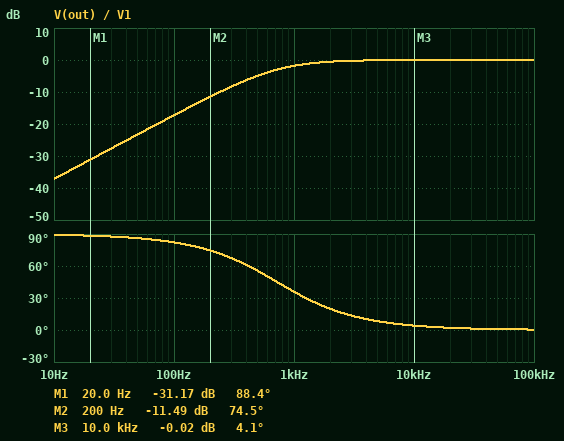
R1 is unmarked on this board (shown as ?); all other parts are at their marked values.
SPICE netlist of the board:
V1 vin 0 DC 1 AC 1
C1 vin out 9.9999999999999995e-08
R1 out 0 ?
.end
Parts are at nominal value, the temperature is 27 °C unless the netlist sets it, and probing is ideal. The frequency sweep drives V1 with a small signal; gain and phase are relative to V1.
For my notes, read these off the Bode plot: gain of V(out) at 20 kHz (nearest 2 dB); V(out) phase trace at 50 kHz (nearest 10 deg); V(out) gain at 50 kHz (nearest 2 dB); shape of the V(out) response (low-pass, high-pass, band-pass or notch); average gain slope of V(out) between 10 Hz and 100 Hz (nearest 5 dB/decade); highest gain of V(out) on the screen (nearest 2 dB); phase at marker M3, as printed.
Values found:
0 dB
0 deg
0 dB
high-pass
20 dB/decade
0 dB
4.1 deg
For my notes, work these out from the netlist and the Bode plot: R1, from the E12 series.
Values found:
2.2 kΩ
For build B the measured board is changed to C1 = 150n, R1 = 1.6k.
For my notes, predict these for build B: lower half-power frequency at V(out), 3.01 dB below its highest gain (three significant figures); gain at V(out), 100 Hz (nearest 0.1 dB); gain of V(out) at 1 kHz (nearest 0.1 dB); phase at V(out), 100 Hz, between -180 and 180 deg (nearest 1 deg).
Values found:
663 Hz
-16.5 dB
-1.6 dB
81 deg
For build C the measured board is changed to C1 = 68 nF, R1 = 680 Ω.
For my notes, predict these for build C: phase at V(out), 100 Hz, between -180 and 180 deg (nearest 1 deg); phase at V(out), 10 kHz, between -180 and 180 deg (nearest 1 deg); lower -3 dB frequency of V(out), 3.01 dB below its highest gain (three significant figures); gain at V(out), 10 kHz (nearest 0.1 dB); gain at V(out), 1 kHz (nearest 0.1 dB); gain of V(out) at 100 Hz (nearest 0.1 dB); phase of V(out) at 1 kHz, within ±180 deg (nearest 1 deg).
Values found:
88 deg
19 deg
3.44 kHz
-0.5 dB
-11.1 dB
-30.7 dB
74 deg
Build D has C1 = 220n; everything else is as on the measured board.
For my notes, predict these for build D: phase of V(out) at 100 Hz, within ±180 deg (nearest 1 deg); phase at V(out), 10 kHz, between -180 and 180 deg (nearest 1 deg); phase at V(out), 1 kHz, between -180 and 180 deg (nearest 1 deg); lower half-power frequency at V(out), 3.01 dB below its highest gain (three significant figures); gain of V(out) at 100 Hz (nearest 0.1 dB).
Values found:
73 deg
2 deg
18 deg
329 Hz
-10.7 dB
